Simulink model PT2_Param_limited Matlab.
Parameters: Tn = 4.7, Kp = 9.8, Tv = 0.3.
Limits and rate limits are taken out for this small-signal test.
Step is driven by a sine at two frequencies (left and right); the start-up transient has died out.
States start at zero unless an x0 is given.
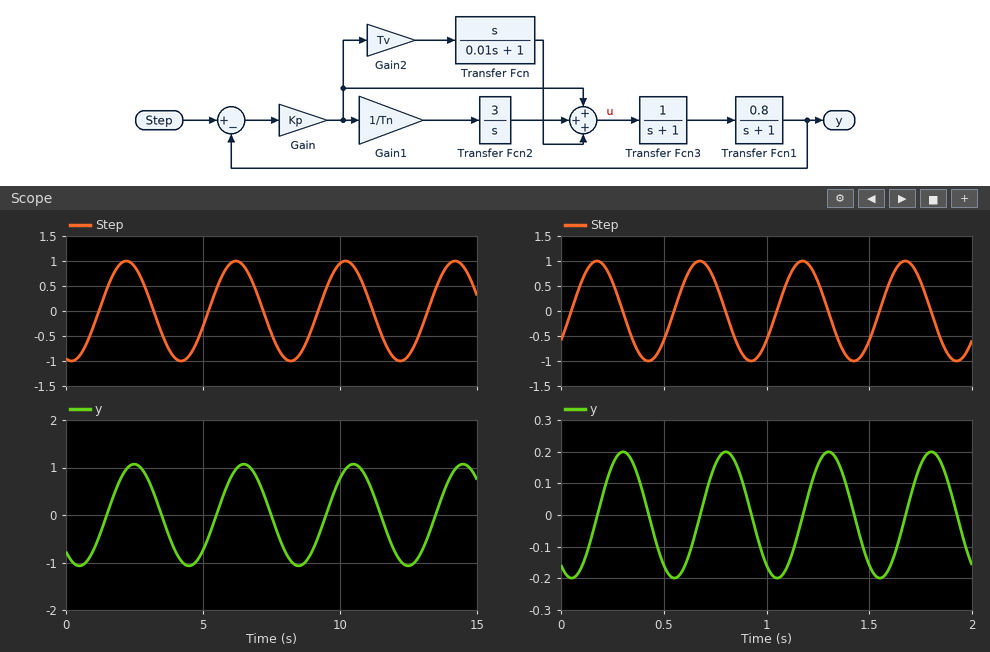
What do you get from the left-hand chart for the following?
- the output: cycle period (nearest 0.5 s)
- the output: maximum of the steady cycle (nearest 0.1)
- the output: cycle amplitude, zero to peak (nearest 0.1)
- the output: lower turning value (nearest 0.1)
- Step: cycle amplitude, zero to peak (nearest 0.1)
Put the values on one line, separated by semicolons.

4.0 s; 1.1; 1.1; -1.1; 1.0
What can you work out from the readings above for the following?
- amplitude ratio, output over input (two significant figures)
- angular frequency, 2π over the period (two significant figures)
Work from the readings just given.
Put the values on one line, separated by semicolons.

1.1; 1.6 rad/s
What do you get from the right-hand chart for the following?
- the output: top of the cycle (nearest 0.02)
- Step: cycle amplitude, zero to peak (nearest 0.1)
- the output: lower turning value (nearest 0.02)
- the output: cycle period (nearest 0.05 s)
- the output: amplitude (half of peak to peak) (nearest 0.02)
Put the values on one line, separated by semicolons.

0.20; 1.0; -0.20; 0.50 s; 0.20
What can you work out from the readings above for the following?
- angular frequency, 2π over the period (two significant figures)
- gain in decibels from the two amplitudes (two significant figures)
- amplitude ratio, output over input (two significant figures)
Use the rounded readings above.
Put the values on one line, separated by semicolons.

13 rad/s; -14 dB; 0.20
